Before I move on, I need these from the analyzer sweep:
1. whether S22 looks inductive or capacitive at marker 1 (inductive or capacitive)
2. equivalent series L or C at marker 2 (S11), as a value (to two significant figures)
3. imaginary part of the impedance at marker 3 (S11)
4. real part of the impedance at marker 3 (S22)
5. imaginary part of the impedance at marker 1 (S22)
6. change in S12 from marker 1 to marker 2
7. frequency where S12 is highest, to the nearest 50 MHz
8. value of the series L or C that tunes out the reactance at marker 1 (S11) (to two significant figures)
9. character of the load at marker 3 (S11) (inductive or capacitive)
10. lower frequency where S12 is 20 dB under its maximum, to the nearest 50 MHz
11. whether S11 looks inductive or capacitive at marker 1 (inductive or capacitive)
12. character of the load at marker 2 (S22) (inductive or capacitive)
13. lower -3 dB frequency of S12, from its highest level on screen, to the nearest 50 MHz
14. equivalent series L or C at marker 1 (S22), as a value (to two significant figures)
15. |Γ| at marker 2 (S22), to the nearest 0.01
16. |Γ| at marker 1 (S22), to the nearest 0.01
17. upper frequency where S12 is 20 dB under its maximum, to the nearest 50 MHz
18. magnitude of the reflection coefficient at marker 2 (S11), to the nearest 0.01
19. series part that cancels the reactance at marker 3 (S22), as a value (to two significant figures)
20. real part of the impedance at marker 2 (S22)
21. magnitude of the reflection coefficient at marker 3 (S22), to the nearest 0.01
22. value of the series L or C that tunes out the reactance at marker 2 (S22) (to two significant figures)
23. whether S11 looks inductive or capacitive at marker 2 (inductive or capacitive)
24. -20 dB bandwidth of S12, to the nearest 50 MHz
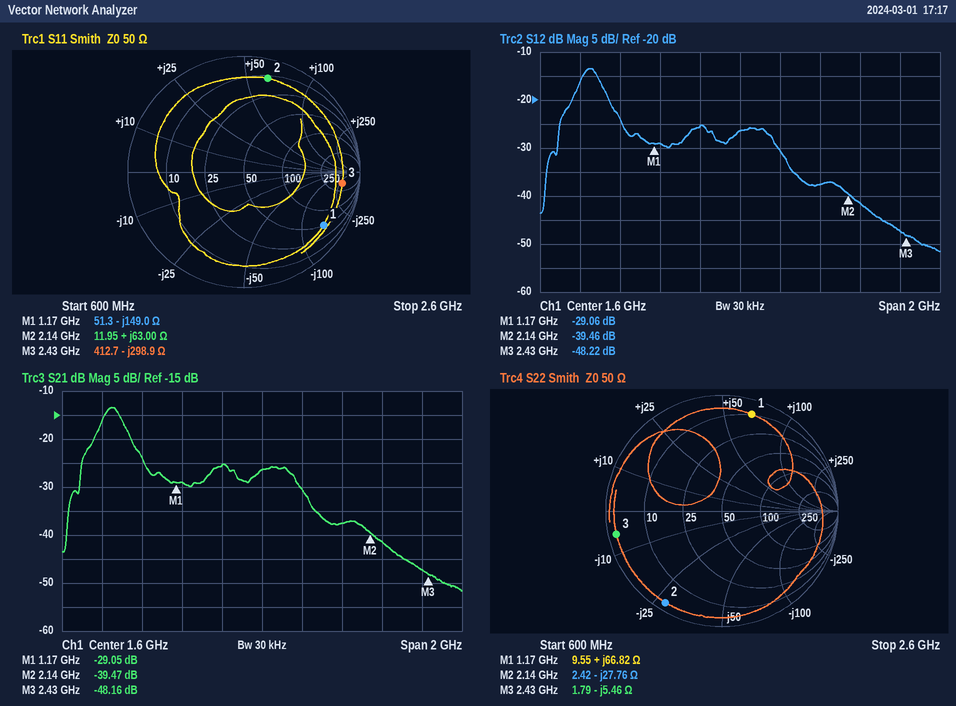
inductive
4.7 nH
-298.9 Ω
1.79 Ω
+66.82 Ω
-10.40 dB
850 MHz
20 nH
capacitive
650 MHz
capacitive
capacitive
800 MHz
9.1 nH
0.93
0.87
1.85 GHz
0.83
360 pH
2.42 Ω
0.93
2.1 nH
inductive
1.20 GHz
